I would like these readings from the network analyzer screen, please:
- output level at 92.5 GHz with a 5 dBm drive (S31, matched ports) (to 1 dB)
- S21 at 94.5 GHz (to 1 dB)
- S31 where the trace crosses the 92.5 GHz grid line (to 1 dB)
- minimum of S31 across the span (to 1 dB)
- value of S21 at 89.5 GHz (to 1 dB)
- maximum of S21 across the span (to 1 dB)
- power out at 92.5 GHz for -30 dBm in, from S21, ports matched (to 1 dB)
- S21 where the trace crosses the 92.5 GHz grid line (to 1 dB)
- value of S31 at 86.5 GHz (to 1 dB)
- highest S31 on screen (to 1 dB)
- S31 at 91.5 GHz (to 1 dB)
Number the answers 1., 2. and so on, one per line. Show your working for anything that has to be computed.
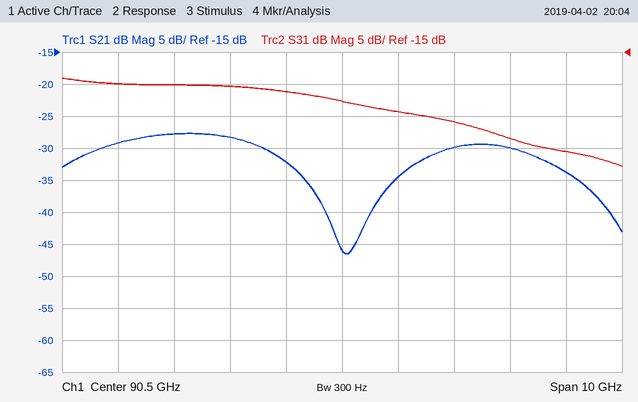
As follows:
1. 5 dBm + (-26 dB) = -21 dBm
2. -34 dB
3. -26 dB
4. -33 dB
5. -32 dB
6. -28 dB
7. -30 dBm + (-30 dB) = -60 dBm
8. -30 dB
9. -20 dB
10. -19 dB
11. -24 dB
